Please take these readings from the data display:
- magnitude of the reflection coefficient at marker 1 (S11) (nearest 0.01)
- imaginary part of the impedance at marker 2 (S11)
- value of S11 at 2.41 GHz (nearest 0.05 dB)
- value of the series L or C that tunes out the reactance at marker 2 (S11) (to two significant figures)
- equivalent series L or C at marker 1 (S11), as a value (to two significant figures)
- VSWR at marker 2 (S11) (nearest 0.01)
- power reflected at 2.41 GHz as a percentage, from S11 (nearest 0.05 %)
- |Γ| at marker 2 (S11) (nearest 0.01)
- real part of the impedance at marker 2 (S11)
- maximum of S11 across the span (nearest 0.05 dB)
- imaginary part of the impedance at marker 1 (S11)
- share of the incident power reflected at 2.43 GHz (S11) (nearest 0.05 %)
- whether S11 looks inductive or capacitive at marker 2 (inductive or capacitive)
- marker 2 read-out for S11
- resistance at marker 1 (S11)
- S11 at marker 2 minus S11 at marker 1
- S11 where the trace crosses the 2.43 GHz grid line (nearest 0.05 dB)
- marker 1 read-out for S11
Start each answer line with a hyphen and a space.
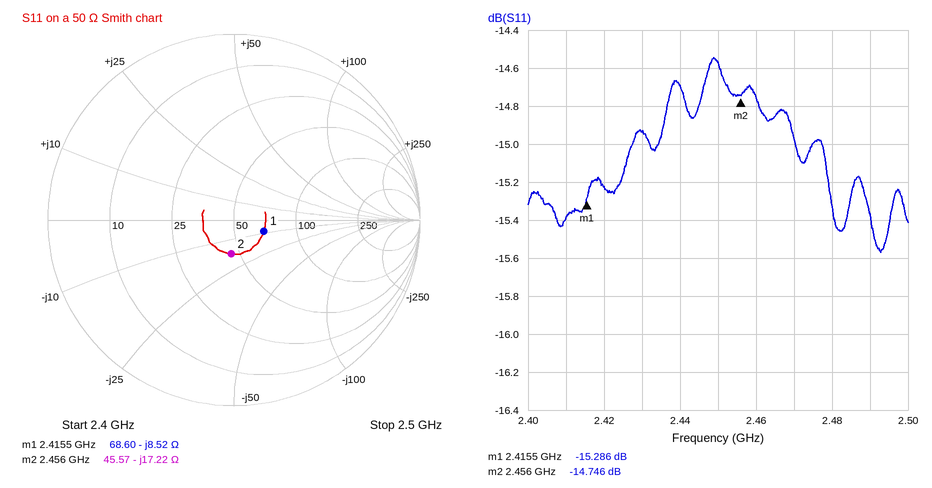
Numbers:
- 0.17
- -17.22 Ω
- -15.40 dB
- 1.1 nH
- 7.7 pF
- 1.45
- 2.90 %
- 0.18
- 45.57 Ω
- -14.55 dB
- -8.52 Ω
- 3.20 %
- capacitive
- -14.746 dB
- 68.60 Ω
- 0.540 dB
- -14.95 dB
- -15.286 dB
